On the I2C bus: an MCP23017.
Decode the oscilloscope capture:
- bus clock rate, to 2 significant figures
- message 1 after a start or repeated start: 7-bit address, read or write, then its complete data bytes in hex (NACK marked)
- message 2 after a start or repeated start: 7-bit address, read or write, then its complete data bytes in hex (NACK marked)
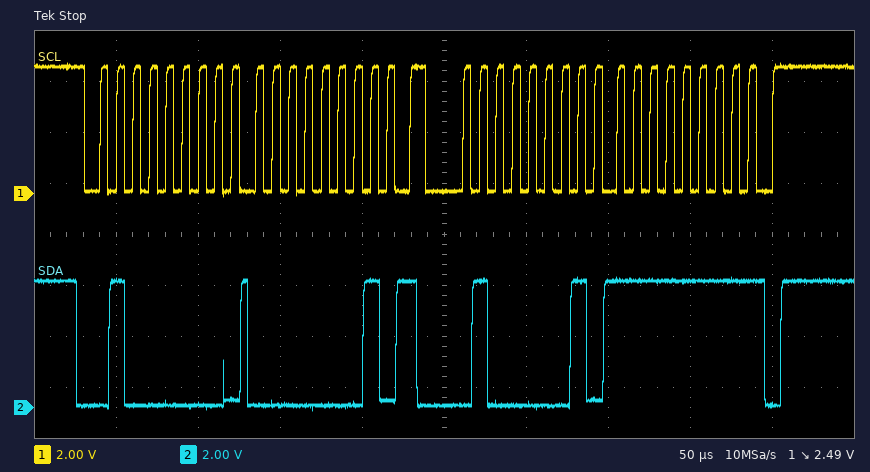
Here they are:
100 kHz
0x20 write: 01
0x20 read: FF NACK
